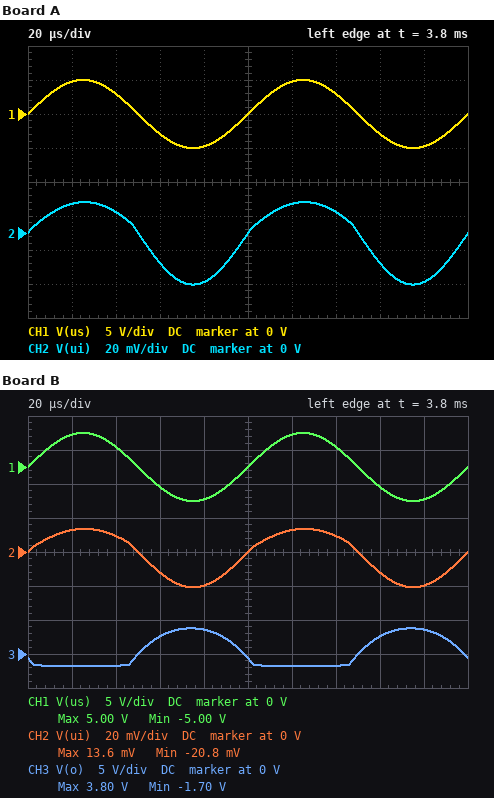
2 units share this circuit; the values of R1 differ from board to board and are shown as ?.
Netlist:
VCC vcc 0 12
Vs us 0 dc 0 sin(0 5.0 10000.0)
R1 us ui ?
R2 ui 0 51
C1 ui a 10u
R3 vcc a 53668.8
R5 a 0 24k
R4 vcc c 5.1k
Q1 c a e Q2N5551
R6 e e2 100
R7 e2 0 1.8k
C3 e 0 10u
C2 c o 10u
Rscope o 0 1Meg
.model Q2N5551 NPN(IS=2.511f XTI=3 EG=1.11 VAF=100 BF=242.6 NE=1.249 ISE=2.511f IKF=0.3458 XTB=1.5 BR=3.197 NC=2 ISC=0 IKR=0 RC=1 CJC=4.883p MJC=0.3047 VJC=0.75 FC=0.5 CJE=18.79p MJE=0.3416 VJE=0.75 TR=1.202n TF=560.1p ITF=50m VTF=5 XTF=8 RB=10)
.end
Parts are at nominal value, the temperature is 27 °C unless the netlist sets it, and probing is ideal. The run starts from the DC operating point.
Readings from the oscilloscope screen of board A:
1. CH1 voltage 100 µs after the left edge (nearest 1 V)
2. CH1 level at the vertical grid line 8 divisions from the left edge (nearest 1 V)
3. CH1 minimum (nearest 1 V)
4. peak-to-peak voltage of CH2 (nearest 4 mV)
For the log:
0 V
-3 V
-5 V
48 mV
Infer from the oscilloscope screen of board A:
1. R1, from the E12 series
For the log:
8.2 kΩ
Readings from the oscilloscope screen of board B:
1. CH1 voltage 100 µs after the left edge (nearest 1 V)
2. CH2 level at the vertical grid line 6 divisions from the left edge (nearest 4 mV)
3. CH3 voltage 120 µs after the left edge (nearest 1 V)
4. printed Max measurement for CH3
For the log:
0 V
12 mV
-2 V
3.80 V
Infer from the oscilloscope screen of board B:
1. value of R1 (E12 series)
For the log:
12 kΩ
